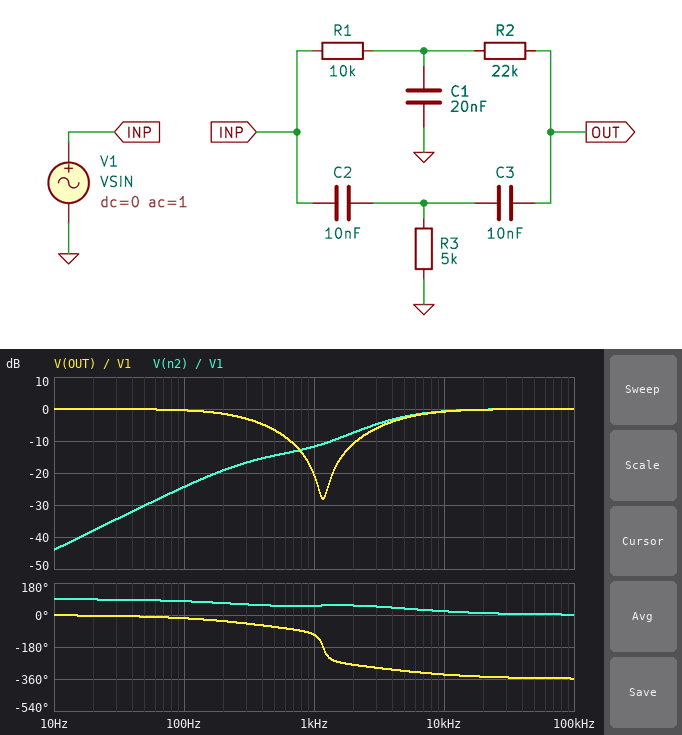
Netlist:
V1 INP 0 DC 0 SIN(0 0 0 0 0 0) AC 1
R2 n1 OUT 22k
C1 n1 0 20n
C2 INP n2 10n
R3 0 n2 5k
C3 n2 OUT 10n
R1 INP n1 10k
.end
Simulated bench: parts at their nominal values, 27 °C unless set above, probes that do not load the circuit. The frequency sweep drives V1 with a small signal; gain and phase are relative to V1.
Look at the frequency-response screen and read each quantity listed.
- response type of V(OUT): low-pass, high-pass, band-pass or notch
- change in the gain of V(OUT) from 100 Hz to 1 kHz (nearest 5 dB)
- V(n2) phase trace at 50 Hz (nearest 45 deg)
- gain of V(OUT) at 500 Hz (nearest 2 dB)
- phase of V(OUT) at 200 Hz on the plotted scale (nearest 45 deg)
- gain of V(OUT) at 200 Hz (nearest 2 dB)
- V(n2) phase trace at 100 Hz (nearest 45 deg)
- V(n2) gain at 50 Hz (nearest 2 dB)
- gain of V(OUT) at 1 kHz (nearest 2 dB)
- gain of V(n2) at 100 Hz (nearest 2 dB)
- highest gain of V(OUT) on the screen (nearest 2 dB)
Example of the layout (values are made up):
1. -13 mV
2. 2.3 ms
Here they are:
1. notch
2. -20 dB
3. 90 deg
4. -6 dB
5. -45 deg
6. -2 dB
7. 90 deg
8. -30 dB
9. -20 dB
10. -24 dB
11. 0 dB
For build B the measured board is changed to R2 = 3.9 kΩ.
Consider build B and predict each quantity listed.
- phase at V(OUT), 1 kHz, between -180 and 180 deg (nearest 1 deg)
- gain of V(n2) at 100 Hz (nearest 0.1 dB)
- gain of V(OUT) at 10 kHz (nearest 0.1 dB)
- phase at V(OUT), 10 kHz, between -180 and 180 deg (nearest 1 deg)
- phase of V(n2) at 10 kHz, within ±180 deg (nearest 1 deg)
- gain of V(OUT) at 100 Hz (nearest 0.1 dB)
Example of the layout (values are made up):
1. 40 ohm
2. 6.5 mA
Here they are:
1. -62 deg
2. -24.2 dB
3. -4.2 dB
4. 47 deg
5. 27 deg
6. -0.2 dB
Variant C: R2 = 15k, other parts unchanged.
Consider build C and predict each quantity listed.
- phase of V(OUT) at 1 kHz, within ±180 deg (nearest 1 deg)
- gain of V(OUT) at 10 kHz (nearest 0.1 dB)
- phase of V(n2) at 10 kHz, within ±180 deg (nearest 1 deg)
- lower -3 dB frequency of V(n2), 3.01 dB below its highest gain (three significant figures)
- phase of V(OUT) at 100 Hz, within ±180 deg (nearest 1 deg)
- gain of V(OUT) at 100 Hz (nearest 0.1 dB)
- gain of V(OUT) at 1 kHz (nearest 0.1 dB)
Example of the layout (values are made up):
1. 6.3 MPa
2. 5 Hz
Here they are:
1. -89 deg
2. -1.1 dB
3. 22 deg
4. 4.77 kHz
5. -16 deg
6. -0.3 dB
7. -15.6 dB
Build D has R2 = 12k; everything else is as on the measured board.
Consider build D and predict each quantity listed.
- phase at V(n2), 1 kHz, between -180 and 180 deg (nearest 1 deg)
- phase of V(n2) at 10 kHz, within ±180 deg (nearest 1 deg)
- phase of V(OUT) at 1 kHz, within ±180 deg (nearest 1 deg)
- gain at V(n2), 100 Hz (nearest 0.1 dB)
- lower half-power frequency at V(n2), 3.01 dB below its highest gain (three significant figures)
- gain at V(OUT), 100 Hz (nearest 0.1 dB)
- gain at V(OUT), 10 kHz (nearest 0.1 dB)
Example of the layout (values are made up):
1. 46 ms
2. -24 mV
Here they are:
1. 47 deg
2. 23 deg
3. -81 deg
4. -24.3 dB
5. 5.15 kHz
6. -0.3 dB
7. -1.3 dB
